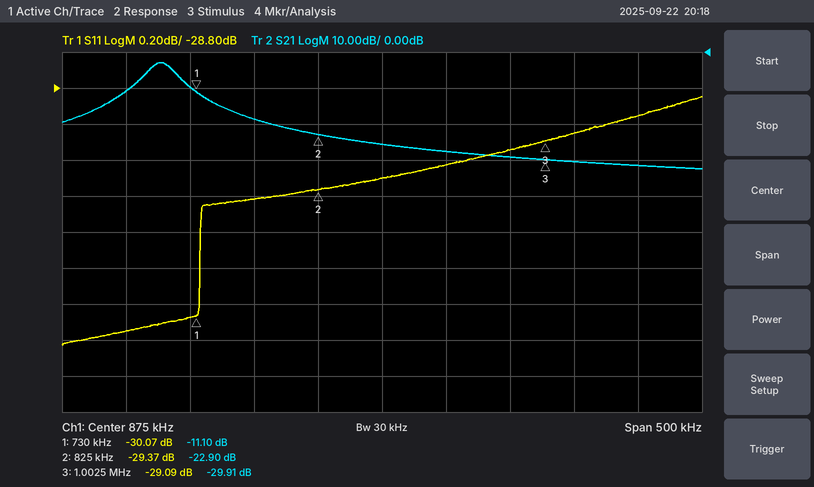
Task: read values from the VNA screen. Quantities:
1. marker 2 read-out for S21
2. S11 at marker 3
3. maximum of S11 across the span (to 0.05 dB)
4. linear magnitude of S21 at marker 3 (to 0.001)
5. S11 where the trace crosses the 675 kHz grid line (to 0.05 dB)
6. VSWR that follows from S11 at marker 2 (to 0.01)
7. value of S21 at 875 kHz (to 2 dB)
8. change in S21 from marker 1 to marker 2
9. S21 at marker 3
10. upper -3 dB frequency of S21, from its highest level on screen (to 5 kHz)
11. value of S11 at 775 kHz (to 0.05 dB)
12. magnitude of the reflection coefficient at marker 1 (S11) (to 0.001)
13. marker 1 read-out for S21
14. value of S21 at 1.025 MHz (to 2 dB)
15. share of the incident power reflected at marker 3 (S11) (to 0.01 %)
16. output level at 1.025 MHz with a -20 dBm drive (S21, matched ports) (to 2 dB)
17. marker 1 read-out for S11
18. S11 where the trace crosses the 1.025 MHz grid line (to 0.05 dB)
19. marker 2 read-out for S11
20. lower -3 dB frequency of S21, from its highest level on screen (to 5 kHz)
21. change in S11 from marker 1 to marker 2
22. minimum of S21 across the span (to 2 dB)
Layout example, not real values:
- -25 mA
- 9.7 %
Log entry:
- -22.90 dB
- -29.09 dB
- -28.85 dB
- 0.032
- -30.15 dB
- 1.07
- -26 dB
- -11.80 dB
- -29.91 dB
- 715 kHz
- -29.40 dB
- 0.031
- -11.10 dB
- -30 dB
- 0.12 %
- -50 dBm
- -30.07 dB
- -29.05 dB
- -29.37 dB
- 690 kHz
- 0.70 dB
- -32 dB
